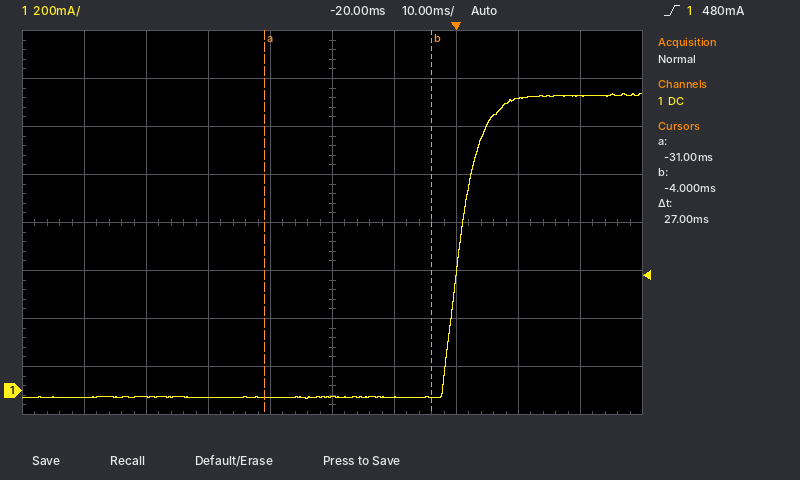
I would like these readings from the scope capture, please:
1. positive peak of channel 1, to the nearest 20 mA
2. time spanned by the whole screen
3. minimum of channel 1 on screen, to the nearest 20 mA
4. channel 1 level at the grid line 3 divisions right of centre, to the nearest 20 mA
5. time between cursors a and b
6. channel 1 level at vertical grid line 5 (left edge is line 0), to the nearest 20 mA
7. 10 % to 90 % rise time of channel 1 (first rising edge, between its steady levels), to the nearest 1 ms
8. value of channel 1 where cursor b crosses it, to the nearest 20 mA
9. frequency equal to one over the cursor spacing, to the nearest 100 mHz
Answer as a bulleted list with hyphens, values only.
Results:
- 1.24 A
- 100 ms
- -40 mA
- 1.22 A
- 27 ms
- -20 mA
- 7 ms
- -20 mA
- 37.0 Hz
